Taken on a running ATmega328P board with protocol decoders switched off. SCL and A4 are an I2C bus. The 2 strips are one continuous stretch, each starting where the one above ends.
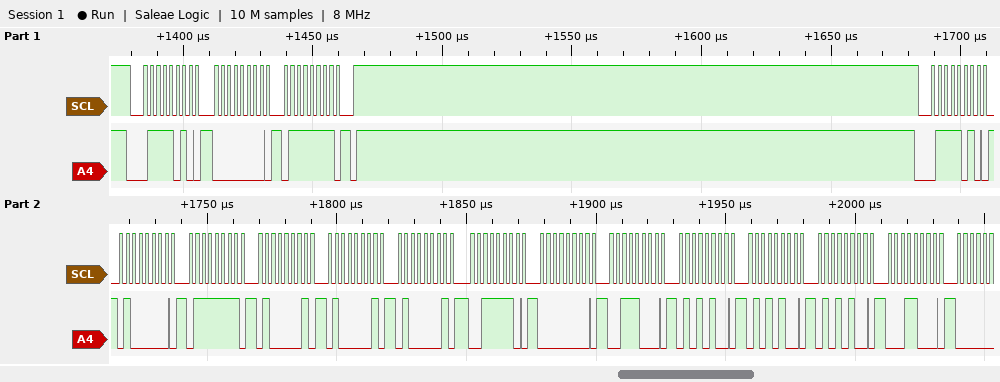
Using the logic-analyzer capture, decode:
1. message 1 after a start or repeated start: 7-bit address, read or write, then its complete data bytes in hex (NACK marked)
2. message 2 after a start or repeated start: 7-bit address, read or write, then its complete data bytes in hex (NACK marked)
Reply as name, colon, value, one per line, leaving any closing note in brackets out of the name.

message 1 after a start or repeated start: 7-bit address, read or write, then its complete data bytes in hex: 0x3D write: 00 7F
message 2 after a start or repeated start: 7-bit address, read or write, then its complete data bytes in hex: 0x3D write: 40 7F 41 41 41 3E 00 38 54 54 54 18
